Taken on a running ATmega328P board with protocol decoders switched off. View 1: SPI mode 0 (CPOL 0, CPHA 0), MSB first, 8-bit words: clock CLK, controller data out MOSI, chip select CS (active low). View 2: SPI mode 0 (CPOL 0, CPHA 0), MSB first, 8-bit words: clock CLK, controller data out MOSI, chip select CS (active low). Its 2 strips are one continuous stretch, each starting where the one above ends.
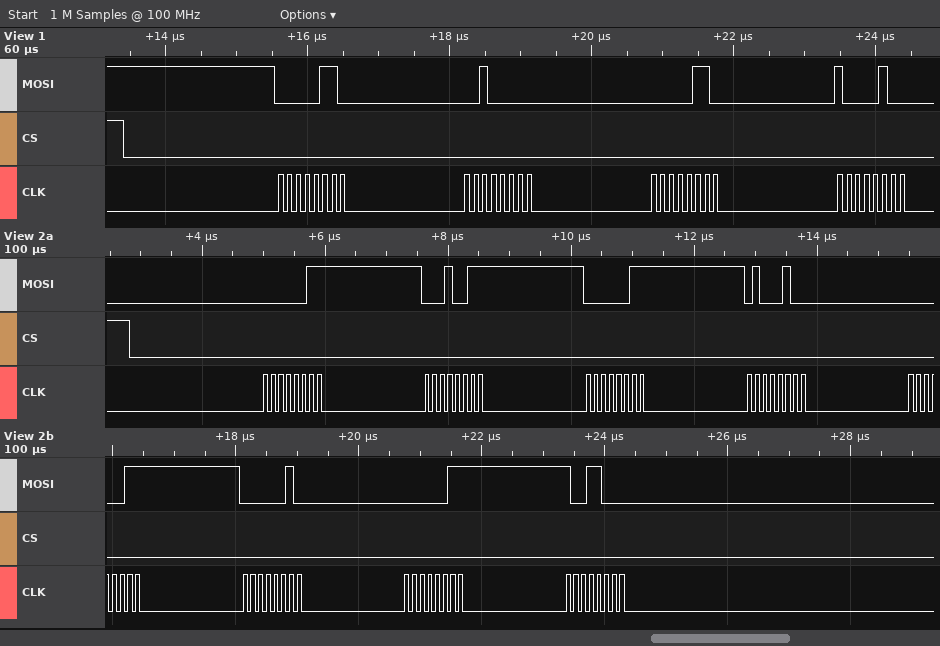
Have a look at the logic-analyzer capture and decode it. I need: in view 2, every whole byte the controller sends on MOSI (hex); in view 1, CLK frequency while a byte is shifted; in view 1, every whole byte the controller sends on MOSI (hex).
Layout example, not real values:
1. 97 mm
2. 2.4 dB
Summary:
1. 03 13 03 44 03 02 03 98
2. 8 MHz
3. 0x06 0x20 0x06 0x84
